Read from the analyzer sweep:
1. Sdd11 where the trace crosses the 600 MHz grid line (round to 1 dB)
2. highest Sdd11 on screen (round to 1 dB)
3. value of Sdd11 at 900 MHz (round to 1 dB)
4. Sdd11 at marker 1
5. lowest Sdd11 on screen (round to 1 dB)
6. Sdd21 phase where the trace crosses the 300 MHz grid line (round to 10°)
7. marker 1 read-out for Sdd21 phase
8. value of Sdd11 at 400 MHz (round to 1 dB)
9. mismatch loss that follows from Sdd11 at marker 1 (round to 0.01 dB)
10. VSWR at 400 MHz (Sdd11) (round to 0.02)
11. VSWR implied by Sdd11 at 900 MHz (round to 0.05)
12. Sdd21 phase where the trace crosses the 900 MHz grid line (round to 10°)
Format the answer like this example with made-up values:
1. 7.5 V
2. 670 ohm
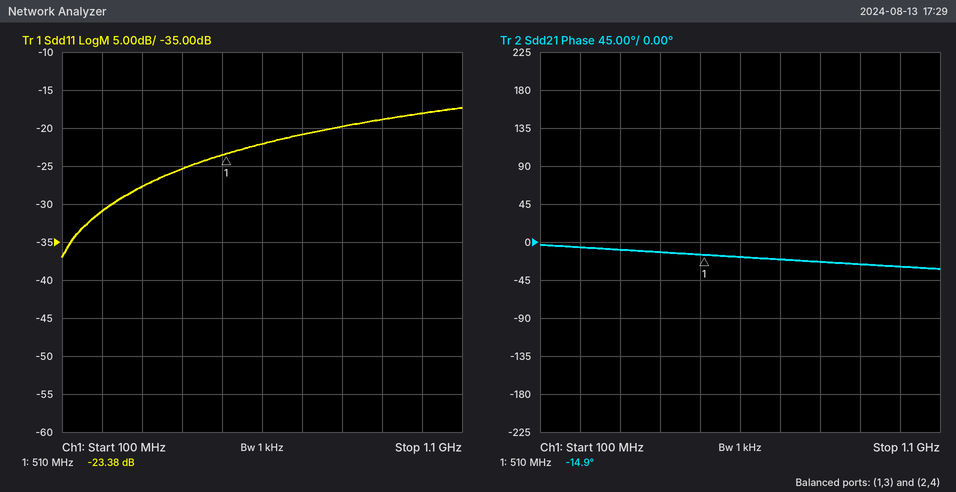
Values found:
1. -22 dB
2. -17 dB
3. -19 dB
4. -23.38 dB
5. -37 dB
6. -10°
7. -14.9°
8. -25 dB
9. 0.02 dB
10. 1.12
11. 1.25
12. -30°
